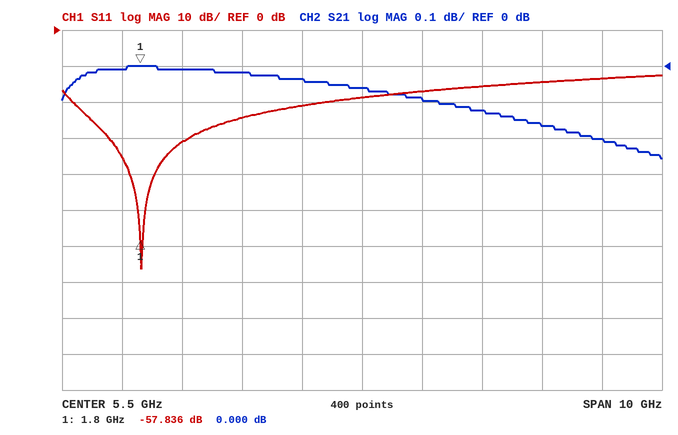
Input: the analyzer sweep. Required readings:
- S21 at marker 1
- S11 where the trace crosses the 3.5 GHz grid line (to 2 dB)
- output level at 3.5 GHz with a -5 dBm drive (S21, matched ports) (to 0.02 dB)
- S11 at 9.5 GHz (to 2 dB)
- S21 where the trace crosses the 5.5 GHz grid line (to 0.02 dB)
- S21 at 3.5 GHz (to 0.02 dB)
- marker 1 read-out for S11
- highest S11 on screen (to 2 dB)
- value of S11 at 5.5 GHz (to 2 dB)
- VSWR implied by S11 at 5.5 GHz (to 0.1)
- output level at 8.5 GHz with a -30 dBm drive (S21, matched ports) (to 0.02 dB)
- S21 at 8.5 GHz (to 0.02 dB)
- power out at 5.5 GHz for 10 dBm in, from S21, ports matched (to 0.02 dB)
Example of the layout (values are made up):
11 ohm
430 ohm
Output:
0.000 dB
-24 dB
-5.02 dBm
-14 dB
-0.06 dB
-0.02 dB
-57.836 dB
-12 dB
-18 dB
1.3
-30.16 dBm
-0.16 dB
9.94 dBm
